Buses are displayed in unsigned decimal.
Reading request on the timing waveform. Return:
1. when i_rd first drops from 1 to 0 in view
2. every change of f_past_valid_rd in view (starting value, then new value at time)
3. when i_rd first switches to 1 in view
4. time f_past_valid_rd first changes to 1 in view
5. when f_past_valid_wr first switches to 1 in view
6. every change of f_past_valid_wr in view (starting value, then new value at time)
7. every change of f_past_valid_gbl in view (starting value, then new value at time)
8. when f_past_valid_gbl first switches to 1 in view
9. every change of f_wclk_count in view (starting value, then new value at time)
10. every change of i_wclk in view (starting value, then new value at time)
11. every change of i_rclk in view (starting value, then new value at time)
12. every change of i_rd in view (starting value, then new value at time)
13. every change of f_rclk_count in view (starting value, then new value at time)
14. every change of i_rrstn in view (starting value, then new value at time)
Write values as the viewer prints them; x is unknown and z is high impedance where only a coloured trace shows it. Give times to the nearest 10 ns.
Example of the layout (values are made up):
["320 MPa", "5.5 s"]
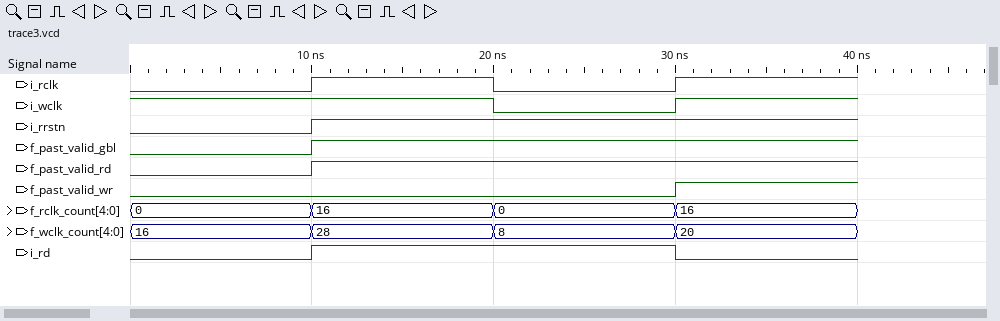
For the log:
["30 ns", "0, 1 at 10 ns", "10 ns", "10 ns", "30 ns", "0, 1 at 30 ns", "0, 1 at 10 ns", "10 ns", "16, 28 at 10 ns, 8 at 20 ns, 20 at 30 ns", "1, 0 at 20 ns, 1 at 30 ns", "0, 1 at 10 ns, 0 at 20 ns, 1 at 30 ns", "0, 1 at 10 ns, 0 at 30 ns", "0, 16 at 10 ns, 0 at 20 ns, 16 at 30 ns", "0, 1 at 10 ns"]
